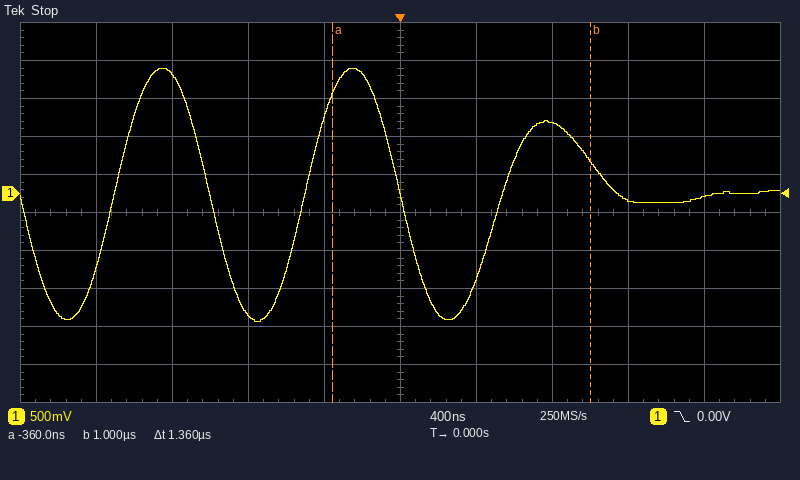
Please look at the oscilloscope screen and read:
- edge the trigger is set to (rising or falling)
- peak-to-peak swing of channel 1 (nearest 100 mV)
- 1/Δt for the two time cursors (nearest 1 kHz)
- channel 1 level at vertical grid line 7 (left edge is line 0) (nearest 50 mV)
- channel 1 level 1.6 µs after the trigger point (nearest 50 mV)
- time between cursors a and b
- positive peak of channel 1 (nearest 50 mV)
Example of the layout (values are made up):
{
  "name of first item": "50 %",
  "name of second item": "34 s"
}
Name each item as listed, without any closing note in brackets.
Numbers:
{
  "edge the trigger is set to": "falling",
  "peak-to-peak swing of channel 1": "3.30 V",
  "1/Δt for the two time cursors": "735 kHz",
  "channel 1 level at vertical grid line 7 (left edge is line 0)": "950 mV",
  "channel 1 level 1.6 µs after the trigger point": "-50 mV",
  "time between cursors a and b": "1.36 µs",
  "positive peak of channel 1": "1.65 V"
}
